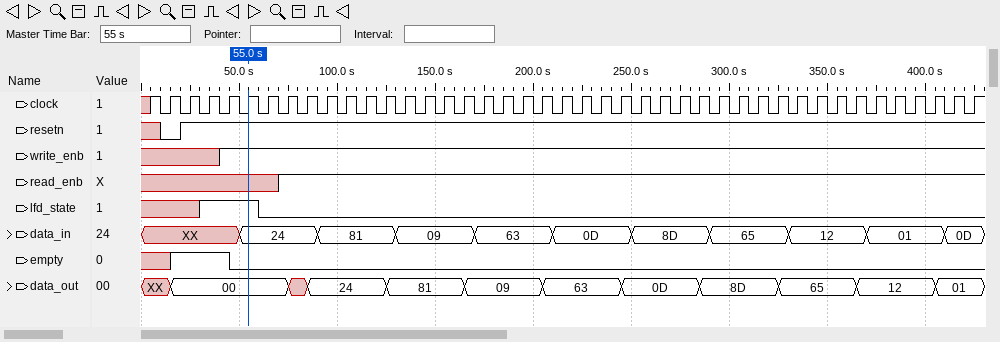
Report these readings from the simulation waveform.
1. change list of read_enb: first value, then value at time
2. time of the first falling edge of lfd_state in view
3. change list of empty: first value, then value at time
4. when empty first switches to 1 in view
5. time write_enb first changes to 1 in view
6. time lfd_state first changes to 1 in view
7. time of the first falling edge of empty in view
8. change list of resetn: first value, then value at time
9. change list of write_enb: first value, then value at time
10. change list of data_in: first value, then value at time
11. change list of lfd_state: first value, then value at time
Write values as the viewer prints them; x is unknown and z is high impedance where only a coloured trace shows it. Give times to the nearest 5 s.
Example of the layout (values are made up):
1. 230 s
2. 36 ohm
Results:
1. x, 1 at 70 s
2. 60 s
3. x, 1 at 15 s, 0 at 45 s
4. 15 s
5. 40 s
6. 30 s
7. 45 s
8. x, 0 at 10 s, 1 at 20 s
9. x, 1 at 40 s
10. XX, 24 at 50 s, 81 at 90 s, 09 at 130 s, 63 at 170 s, 0D at 210 s, 8D at 250 s, 65 at 290 s, 12 at 330 s, 01 at 370 s, 0D at 410 s
11. x, 1 at 30 s, 0 at 60 s
